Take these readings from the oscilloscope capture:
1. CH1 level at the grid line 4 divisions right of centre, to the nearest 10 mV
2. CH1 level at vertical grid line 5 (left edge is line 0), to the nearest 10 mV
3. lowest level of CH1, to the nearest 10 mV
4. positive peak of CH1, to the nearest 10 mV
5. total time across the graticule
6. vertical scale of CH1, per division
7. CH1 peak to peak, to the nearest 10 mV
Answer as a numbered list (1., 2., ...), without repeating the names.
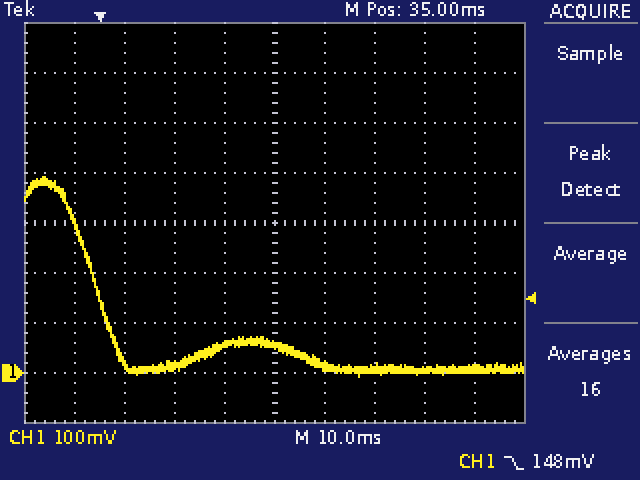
1. 10 mV
2. 60 mV
3. -10 mV
4. 390 mV
5. 100 ms
6. 100 mV
7. 400 mV
